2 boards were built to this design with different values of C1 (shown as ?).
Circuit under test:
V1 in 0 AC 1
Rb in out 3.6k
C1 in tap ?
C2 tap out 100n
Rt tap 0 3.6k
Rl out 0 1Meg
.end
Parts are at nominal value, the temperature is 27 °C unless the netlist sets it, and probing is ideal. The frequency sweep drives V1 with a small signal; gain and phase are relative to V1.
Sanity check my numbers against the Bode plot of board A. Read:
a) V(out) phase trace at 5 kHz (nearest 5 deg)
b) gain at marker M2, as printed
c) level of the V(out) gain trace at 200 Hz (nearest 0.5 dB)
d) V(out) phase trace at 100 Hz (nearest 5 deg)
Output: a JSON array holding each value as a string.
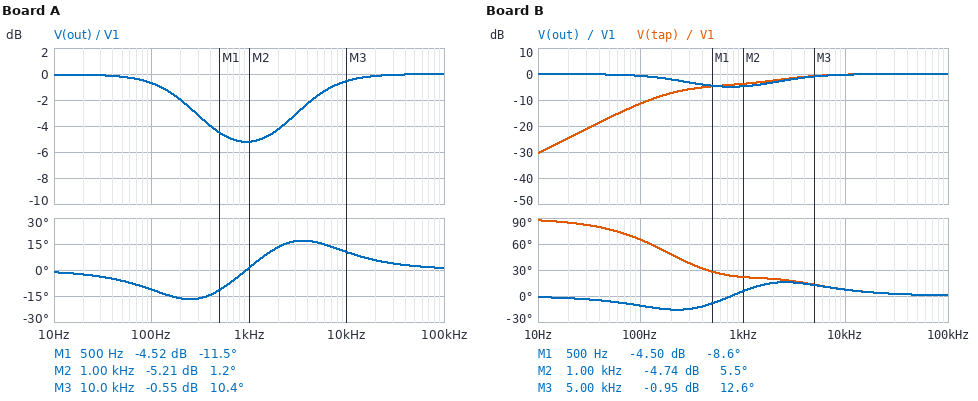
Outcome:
["15 deg", "-5.21 dB", "-2.0 dB", "-10 deg"]
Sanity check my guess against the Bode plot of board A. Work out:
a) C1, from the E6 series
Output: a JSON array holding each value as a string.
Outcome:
["22 nF"]
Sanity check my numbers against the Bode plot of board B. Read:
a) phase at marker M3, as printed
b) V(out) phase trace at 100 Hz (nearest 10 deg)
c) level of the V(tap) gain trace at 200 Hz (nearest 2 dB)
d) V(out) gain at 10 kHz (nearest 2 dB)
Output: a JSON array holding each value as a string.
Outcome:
["12.6 deg", "-10 deg", "-8 dB", "0 dB"]
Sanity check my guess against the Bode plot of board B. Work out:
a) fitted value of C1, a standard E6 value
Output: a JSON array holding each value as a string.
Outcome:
["33 nF"]
